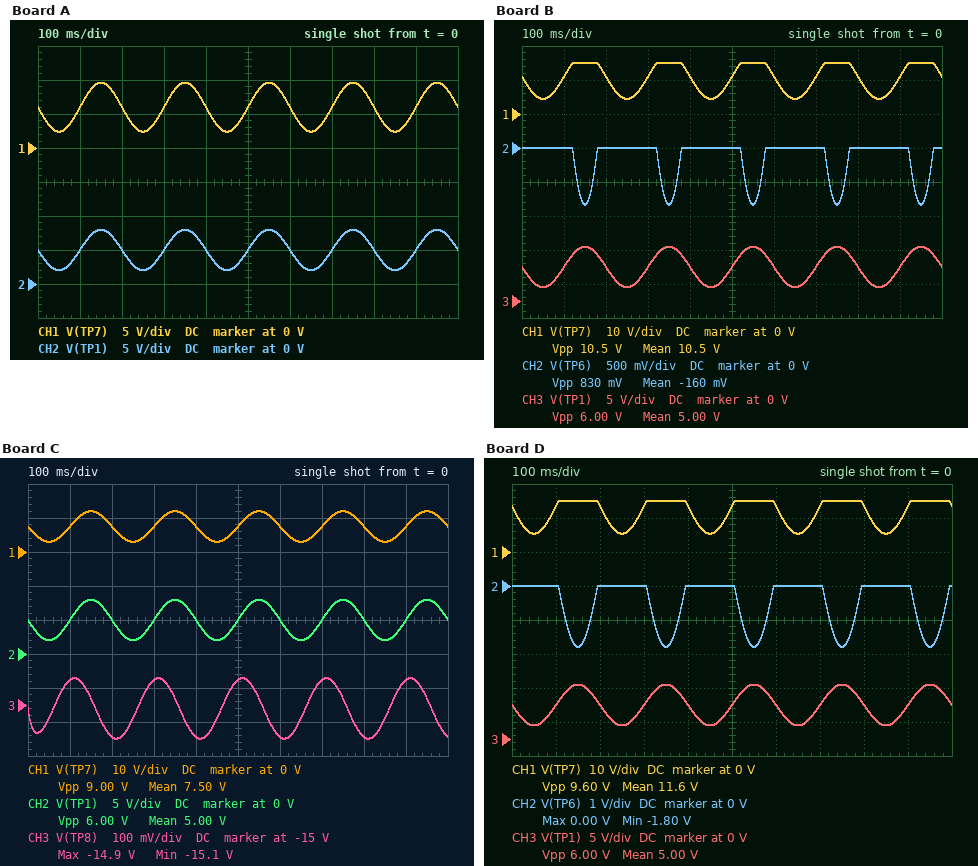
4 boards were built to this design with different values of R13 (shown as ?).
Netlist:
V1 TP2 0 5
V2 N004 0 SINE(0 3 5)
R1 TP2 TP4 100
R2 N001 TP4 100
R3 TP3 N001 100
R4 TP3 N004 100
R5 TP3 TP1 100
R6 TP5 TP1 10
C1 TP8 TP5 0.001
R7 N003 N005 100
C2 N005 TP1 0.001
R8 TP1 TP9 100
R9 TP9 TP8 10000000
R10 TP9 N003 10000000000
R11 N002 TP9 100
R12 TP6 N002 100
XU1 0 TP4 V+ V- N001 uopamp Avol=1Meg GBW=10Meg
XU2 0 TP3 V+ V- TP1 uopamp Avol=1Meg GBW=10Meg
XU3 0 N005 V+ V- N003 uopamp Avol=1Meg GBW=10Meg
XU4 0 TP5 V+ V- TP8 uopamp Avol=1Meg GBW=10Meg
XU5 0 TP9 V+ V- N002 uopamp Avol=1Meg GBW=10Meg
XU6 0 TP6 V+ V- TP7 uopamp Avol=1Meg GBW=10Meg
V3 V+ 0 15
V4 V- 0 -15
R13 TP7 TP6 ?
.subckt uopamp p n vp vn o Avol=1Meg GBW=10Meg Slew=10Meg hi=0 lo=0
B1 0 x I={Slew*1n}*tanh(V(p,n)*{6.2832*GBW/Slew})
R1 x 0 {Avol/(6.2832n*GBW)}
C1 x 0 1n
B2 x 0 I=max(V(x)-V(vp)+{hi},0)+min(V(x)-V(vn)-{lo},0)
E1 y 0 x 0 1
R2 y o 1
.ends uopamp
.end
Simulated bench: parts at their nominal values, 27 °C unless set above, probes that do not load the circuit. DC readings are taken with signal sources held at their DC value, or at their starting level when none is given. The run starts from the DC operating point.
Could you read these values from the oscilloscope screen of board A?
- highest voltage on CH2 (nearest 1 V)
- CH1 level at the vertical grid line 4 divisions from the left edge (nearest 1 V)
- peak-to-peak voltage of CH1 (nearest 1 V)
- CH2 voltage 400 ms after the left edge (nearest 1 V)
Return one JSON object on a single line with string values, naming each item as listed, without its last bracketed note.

{"highest voltage on CH2": "8 V", "CH1 level at the vertical grid line 4 divisions from the left edge": "6 V", "peak-to-peak voltage of CH1": "7 V", "CH2 voltage 400 ms after the left edge": "5 V"}
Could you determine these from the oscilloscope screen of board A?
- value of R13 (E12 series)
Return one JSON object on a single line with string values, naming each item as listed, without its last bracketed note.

{"value of R13": "120 Ω"}
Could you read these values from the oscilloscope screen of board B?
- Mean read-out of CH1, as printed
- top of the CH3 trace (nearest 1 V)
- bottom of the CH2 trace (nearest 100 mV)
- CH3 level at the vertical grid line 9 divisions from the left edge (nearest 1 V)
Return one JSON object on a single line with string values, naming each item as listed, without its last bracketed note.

{"Mean read-out of CH1, as printed": "10.5 V", "top of the CH3 trace": "8 V", "bottom of the CH2 trace": "-800 mV", "CH3 level at the vertical grid line 9 divisions from the left edge": "5 V"}
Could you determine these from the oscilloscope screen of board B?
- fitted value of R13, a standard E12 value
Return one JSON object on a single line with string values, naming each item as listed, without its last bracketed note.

{"fitted value of R13, a standard E12 value": "220 Ω"}
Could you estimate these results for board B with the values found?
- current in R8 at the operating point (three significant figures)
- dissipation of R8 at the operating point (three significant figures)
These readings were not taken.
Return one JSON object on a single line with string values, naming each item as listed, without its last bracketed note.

{"current in R8 at the operating point": "50.0 mA", "dissipation of R8 at the operating point": "250 mW"}
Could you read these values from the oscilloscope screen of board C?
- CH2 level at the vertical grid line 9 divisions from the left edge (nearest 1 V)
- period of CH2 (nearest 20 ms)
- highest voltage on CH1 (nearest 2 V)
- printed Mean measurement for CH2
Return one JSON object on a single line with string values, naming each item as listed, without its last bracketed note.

{"CH2 level at the vertical grid line 9 divisions from the left edge": "5 V", "period of CH2": "200 ms", "highest voltage on CH1": "12 V", "printed Mean measurement for CH2": "5.00 V"}
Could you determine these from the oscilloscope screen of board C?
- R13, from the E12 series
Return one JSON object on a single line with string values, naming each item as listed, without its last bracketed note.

{"R13, from the E12 series": "150 Ω"}
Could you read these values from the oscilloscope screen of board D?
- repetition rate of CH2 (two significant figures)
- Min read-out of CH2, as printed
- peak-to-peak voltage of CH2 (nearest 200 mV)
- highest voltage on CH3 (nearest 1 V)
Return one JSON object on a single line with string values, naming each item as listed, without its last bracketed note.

{"repetition rate of CH2": "5.0 Hz", "Min read-out of CH2, as printed": "-1.80 V", "peak-to-peak voltage of CH2": "1.8 V", "highest voltage on CH3": "8 V"}
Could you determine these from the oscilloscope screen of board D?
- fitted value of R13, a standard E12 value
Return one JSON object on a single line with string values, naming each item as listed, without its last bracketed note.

{"fitted value of R13, a standard E12 value": "270 Ω"}
